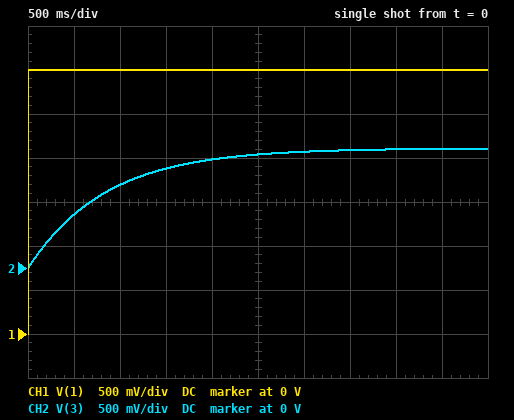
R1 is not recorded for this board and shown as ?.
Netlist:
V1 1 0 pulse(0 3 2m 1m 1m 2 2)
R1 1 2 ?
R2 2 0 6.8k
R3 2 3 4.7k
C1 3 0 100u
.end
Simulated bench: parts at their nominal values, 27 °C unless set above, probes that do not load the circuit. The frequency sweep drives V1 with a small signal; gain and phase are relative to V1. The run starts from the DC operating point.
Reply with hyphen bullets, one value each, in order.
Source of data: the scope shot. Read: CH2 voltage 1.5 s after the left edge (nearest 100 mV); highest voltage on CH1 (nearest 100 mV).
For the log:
- 1.1 V
- 3.0 V
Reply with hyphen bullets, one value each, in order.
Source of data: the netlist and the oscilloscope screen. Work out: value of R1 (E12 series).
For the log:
- 8.2 kΩ
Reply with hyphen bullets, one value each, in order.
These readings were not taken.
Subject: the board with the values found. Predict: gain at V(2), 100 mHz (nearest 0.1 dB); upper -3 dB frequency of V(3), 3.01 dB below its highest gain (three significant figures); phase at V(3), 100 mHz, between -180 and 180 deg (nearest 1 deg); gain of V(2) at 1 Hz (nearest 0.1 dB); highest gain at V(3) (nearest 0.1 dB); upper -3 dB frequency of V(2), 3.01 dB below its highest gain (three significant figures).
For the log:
- -7.6 dB
- 189 mHz
- -28 deg
- -11.6 dB
- -6.9 dB
- 308 mHz
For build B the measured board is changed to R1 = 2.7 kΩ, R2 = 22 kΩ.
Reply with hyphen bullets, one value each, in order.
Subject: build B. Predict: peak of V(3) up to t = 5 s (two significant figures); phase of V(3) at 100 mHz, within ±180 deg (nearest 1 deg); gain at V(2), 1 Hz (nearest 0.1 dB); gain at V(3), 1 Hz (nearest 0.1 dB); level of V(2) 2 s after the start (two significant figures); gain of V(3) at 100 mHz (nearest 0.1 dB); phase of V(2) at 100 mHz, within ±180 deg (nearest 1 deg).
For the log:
- 2.7 V
- -24 deg
- -4.3 dB
- -14.2 dB
- 2.6 V
- -1.8 dB
- -8 deg
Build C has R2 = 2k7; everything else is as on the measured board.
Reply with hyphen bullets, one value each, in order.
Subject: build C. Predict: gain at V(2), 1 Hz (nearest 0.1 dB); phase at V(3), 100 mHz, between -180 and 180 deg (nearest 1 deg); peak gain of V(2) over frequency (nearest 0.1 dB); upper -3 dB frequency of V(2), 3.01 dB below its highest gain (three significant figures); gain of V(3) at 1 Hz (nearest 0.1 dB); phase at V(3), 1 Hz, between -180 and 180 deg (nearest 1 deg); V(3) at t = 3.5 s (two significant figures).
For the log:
- -15.0 dB
- -23 deg
- -12.1 dB
- 1.50 Hz
- -24.9 dB
- -77 deg
- 740 mV
